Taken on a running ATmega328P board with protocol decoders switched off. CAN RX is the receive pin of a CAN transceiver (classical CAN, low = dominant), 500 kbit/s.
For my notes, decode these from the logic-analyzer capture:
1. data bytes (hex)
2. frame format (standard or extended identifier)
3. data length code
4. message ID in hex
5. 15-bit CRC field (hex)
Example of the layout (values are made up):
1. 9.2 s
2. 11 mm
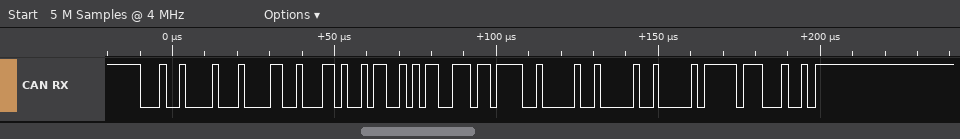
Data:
1. 64 69 65 67 6F 20 20 20
2. standard
3. 8
4. 0x121
5. 0x3FC4
